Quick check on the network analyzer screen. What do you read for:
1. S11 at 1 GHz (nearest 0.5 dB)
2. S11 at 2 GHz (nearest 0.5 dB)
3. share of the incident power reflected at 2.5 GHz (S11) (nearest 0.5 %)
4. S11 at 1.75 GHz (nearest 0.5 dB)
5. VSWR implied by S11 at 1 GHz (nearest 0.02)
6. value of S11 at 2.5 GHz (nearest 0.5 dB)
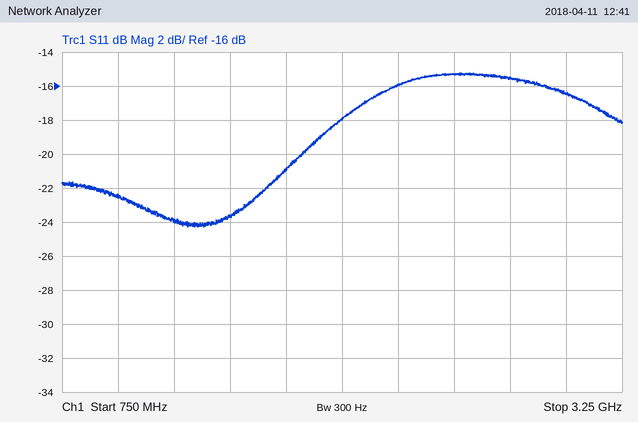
-22.5 dB
-18.0 dB
3.0 %
-21.0 dB
1.16
-15.5 dB
